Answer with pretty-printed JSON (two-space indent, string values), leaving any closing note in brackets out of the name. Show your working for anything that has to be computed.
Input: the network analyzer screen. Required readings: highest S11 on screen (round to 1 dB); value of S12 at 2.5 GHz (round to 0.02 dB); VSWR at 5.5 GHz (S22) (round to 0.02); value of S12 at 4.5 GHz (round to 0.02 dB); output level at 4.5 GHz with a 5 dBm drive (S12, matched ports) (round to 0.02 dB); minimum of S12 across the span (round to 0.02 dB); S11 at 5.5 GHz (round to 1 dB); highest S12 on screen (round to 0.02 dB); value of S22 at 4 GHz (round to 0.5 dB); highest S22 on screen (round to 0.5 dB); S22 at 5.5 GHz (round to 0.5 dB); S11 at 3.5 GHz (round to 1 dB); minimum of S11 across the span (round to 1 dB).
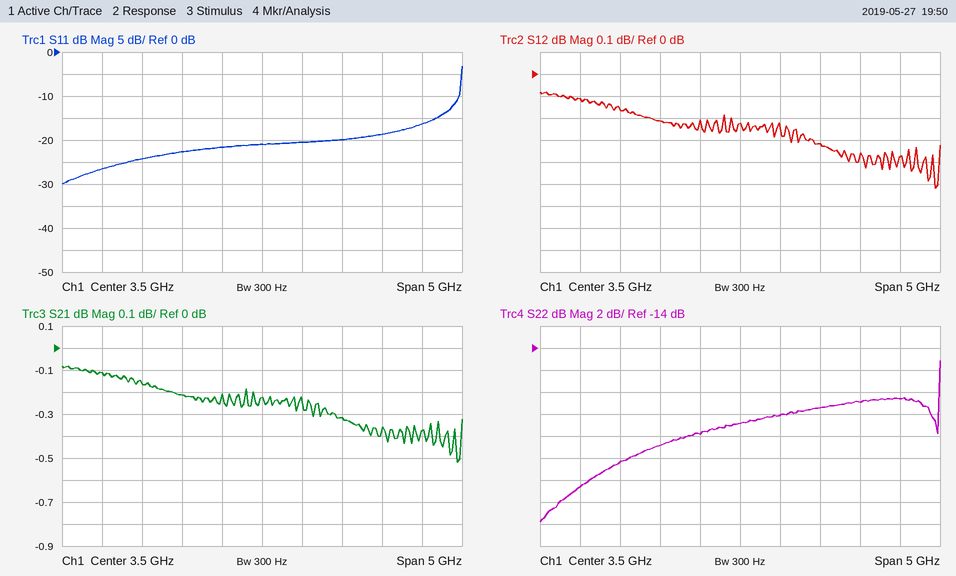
{
  "highest S11 on screen": "-3 dB",
  "value of S12 at 2.5 GHz": "-0.22 dB",
  "VSWR at 5.5 GHz (S22)": "|Γ| = 10^(-18.5/20) = 0.1189; VSWR = (1 + 0.1189)/(1 − 0.1189) ≈ 1.27, so 1.26 to the nearest 0.02",
  "value of S12 at 4.5 GHz": "-0.32 dB",
  "output level at 4.5 GHz with a 5 dBm drive (S12, matched ports)": "5 dBm + (-0.32 dB) = 4.68 dBm",
  "minimum of S12 across the span": "-0.52 dB",
  "S11 at 5.5 GHz": "-16 dB",
  "highest S12 on screen": "-0.08 dB",
  "value of S22 at 4 GHz": "-20.0 dB",
  "highest S22 on screen": "-15.0 dB",
  "S22 at 5.5 GHz": "-18.5 dB",
  "S11 at 3.5 GHz": "-21 dB",
  "minimum of S11 across the span": "-30 dB"
}
